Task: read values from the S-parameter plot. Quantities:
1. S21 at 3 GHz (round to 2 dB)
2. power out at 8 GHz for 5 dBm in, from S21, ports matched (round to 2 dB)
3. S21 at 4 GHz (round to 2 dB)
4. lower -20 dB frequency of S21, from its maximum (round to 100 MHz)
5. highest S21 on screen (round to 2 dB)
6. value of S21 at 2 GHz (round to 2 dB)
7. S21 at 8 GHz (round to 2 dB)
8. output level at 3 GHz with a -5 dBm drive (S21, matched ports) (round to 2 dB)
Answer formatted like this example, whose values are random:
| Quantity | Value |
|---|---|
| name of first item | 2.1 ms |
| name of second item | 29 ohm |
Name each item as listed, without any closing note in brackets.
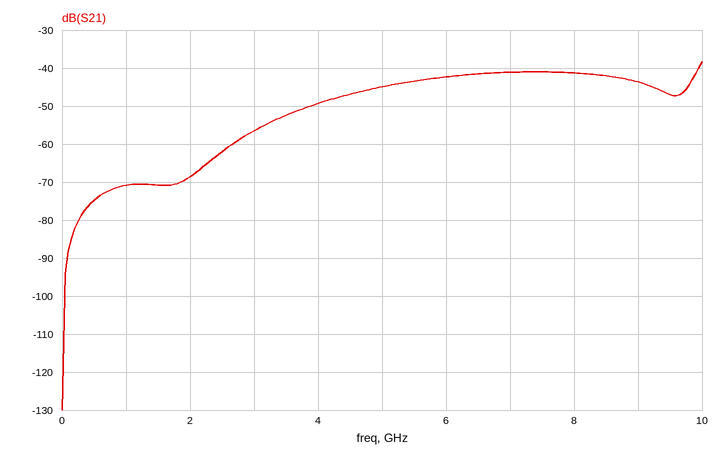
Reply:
| Quantity | Value |
|---|---|
| S21 at 3 GHz | -56 dB |
| power out at 8 GHz for 5 dBm in, from S21, ports matched | -36 dBm |
| S21 at 4 GHz | -50 dB |
| lower -20 dB frequency of S21, from its maximum | 2.8 GHz |
| highest S21 on screen | -38 dB |
| value of S21 at 2 GHz | -68 dB |
| S21 at 8 GHz | -42 dB |
| output level at 3 GHz with a -5 dBm drive (S21, matched ports) | -62 dBm |
